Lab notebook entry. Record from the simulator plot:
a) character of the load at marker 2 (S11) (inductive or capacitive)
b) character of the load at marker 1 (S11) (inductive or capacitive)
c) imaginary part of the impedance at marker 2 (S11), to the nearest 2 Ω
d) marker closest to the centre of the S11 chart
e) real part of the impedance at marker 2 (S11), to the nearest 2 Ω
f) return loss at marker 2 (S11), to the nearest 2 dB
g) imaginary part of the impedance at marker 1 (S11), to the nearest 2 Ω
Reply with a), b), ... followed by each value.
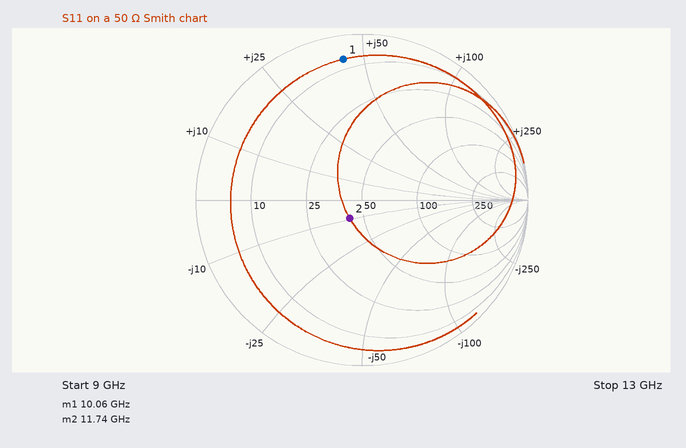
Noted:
a) capacitive
b) inductive
c) -10 Ω
d) marker 2
e) 42 Ω
f) 18 dB
g) +44 Ω
